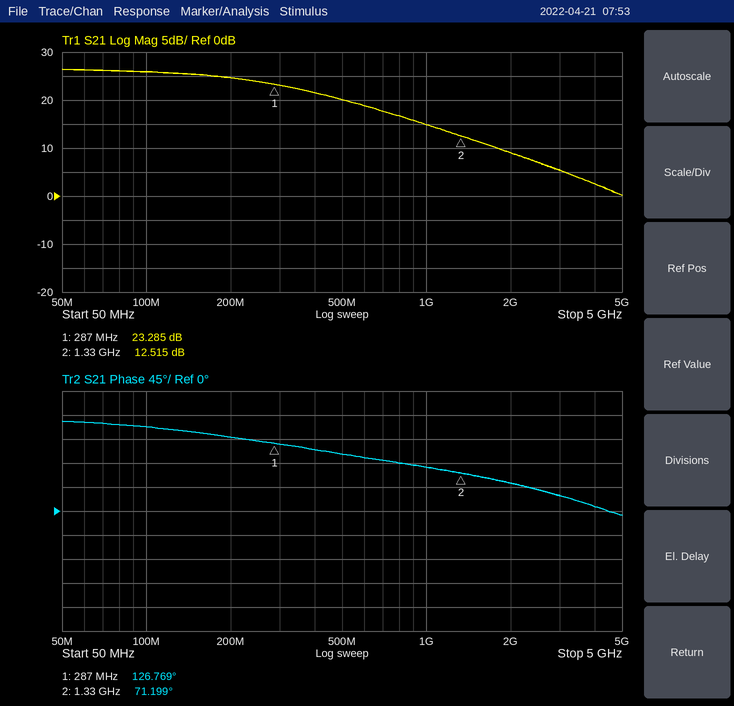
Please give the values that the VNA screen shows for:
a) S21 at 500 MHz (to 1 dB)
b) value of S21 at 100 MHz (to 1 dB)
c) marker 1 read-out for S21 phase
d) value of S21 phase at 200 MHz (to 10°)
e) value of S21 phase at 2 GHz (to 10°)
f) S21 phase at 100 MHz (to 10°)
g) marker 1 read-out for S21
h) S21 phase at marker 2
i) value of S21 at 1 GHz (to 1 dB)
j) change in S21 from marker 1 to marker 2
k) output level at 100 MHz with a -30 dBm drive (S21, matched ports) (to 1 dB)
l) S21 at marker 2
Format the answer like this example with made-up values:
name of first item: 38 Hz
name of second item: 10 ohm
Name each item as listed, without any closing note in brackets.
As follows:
S21 at 500 MHz: 20 dB
value of S21 at 100 MHz: 26 dB
marker 1 read-out for S21 phase: 126.769°
value of S21 phase at 200 MHz: 140°
value of S21 phase at 2 GHz: 50°
S21 phase at 100 MHz: 160°
marker 1 read-out for S21: 23.285 dB
S21 phase at marker 2: 71.199°
value of S21 at 1 GHz: 15 dB
change in S21 from marker 1 to marker 2: -10.770 dB
output level at 100 MHz with a -30 dBm drive (S21, matched ports): -4 dBm
S21 at marker 2: 12.515 dB
